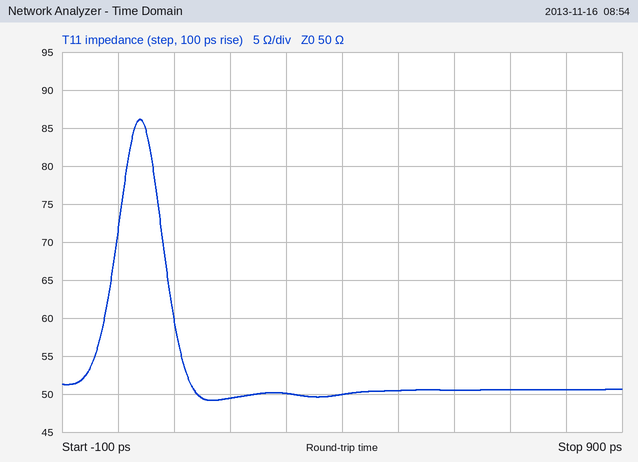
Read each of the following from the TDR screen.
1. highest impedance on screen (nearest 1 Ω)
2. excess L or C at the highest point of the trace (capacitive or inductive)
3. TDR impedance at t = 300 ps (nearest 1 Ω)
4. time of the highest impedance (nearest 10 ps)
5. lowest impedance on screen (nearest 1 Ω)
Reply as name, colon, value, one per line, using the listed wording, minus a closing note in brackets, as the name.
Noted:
highest impedance on screen: 86 Ω
excess L or C at the highest point of the trace: inductive
TDR impedance at t = 300 ps: 50 Ω
time of the highest impedance: 40 ps
lowest impedance on screen: 49 Ω
